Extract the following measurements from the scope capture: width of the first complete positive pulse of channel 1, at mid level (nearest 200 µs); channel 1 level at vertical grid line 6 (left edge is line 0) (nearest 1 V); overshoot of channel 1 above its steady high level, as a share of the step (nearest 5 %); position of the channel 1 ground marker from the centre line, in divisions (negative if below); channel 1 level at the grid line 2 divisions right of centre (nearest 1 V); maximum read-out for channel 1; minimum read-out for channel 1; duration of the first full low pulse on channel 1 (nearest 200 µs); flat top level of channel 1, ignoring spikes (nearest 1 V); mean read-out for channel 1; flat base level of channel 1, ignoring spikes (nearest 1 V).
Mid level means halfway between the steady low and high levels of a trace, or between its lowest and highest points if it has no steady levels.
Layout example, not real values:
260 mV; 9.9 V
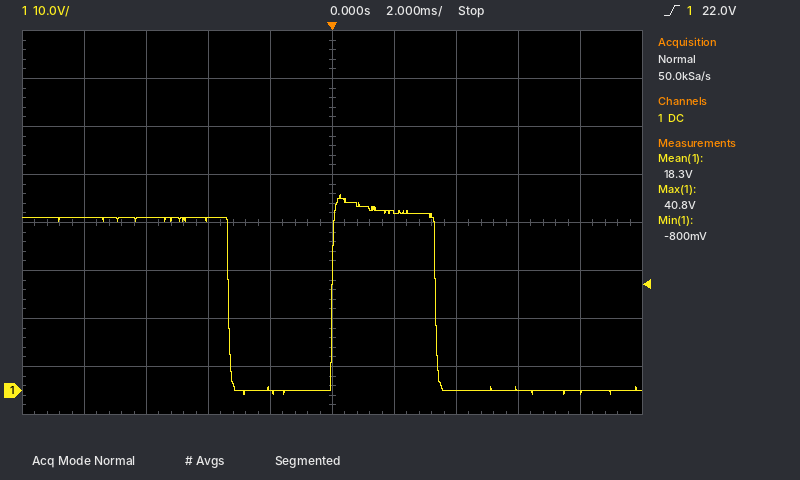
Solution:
3.4 ms; 37 V; 15 %; -3.5 div; 0 V; 40.8 V; -800 mV; 3.4 ms; 36 V; 18.3 V; 0 V
